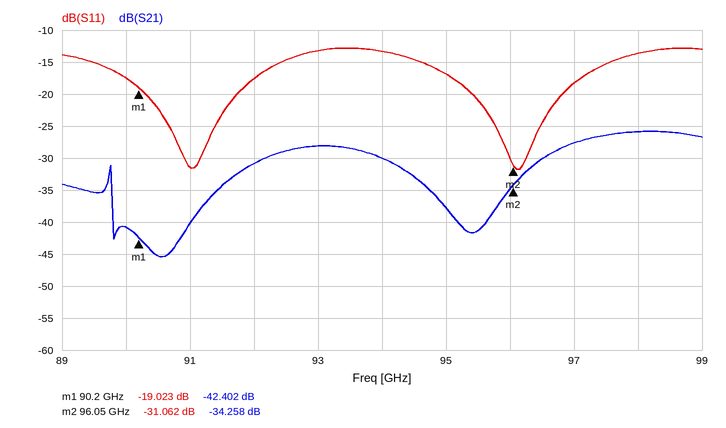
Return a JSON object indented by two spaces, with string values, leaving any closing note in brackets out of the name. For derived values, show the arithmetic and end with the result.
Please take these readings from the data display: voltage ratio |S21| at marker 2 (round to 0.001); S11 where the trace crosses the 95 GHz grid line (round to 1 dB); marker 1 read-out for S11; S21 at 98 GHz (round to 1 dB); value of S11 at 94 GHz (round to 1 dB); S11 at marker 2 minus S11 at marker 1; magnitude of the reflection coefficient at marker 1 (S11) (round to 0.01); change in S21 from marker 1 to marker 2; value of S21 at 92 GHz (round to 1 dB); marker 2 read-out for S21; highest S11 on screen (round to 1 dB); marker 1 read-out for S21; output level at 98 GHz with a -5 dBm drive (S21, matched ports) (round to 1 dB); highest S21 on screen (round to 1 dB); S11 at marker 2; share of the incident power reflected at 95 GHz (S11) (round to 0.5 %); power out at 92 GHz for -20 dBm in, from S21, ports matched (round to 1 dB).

{
  "voltage ratio |S21| at marker 2": "10^(-34.258/20) ≈ 0.019",
  "S11 where the trace crosses the 95 GHz grid line": "-17 dB",
  "marker 1 read-out for S11": "-19.023 dB",
  "S21 at 98 GHz": "-26 dB",
  "value of S11 at 94 GHz": "-13 dB",
  "S11 at marker 2 minus S11 at marker 1": "-31.062 − (-19.023) = -12.039 dB",
  "magnitude of the reflection coefficient at marker 1 (S11)": "10^(-19.023/20) ≈ 0.11",
  "change in S21 from marker 1 to marker 2": "-34.258 − (-42.402) = 8.144 dB",
  "value of S21 at 92 GHz": "-31 dB",
  "marker 2 read-out for S21": "-34.258 dB",
  "highest S11 on screen": "-13 dB",
  "marker 1 read-out for S21": "-42.402 dB",
  "output level at 98 GHz with a -5 dBm drive (S21, matched ports)": "-5 dBm + (-26 dB) = -31 dBm",
  "highest S21 on screen": "-26 dB",
  "S11 at marker 2": "-31.062 dB",
  "share of the incident power reflected at 95 GHz (S11)": "10^(-17/10) ≈ 2.0 %",
  "power out at 92 GHz for -20 dBm in, from S21, ports matched": "-20 dBm + (-31 dB) = -51 dBm"
}
